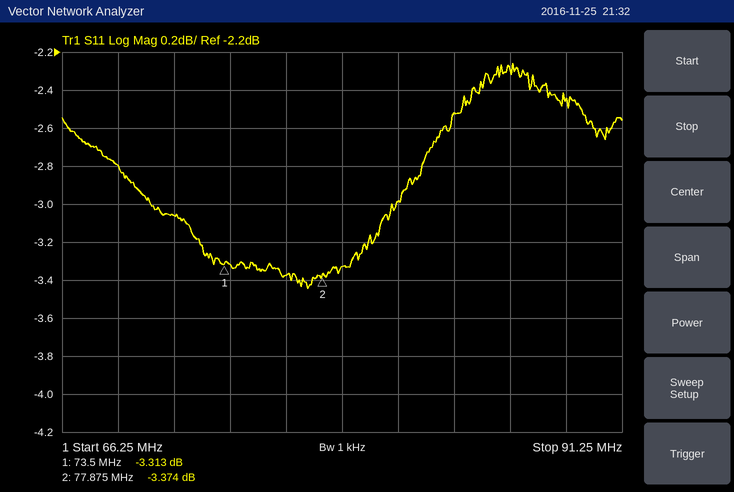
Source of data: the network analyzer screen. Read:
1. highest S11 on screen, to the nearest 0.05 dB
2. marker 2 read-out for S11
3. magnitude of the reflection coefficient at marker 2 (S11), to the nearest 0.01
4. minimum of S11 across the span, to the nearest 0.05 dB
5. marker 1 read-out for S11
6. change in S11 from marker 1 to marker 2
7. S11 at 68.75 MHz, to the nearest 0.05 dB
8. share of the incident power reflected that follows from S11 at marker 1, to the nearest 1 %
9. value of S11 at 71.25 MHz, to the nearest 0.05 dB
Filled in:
-2.25 dB
-3.374 dB
0.68
-3.45 dB
-3.313 dB
-0.061 dB
-2.80 dB
47 %
-3.05 dB
